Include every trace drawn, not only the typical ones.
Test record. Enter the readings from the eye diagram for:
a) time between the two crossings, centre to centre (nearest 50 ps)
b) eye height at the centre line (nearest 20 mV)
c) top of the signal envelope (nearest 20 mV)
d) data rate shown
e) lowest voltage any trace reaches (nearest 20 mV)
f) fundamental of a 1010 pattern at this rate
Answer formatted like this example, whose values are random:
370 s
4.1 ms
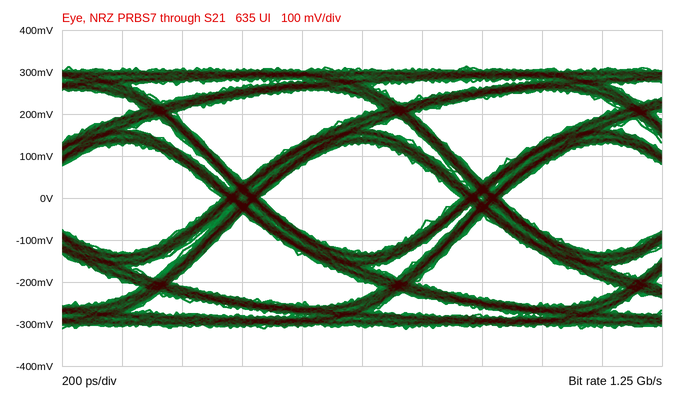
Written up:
800 ps
260 mV
320 mV
1.25 Gb/s
-320 mV
625 MHz
